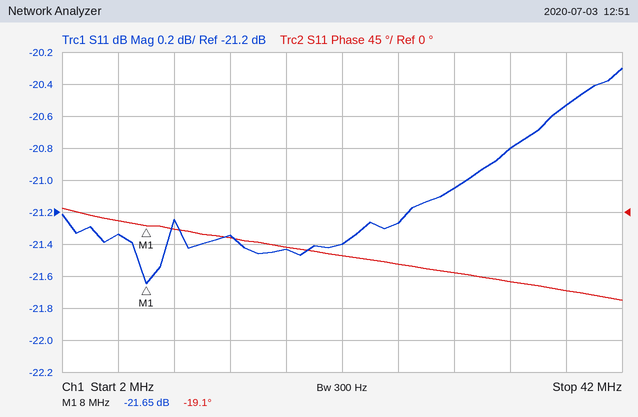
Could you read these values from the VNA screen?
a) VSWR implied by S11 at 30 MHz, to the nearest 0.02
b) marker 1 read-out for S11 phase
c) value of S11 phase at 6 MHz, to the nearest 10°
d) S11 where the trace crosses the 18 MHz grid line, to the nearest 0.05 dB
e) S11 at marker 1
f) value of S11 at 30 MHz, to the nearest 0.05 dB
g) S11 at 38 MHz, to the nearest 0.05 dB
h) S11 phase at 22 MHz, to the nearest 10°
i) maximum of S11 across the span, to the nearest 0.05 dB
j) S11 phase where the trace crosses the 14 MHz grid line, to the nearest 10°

1.20
-19.1°
-10°
-21.45 dB
-21.65 dB
-21.05 dB
-20.55 dB
-60°
-20.30 dB
-40°
